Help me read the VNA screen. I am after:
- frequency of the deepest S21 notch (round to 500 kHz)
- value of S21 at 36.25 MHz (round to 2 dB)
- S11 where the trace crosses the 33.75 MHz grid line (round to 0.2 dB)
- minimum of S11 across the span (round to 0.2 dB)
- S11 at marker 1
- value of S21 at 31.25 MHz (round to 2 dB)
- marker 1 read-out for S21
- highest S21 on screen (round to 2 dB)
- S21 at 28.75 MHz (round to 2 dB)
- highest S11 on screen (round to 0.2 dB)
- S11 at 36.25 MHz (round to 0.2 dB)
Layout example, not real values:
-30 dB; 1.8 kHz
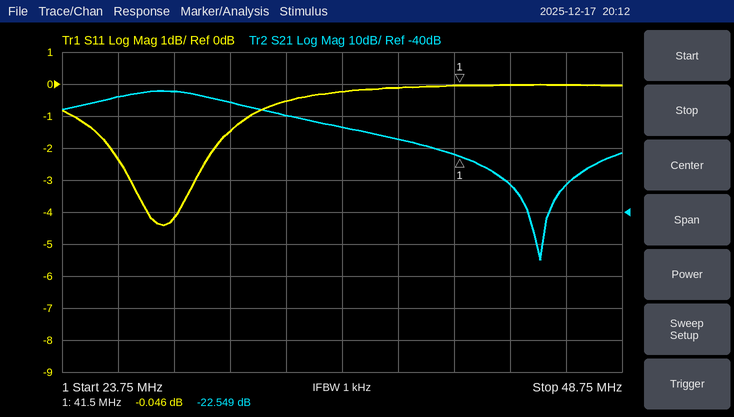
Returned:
45.0 MHz; -14 dB; -0.6 dB; -4.4 dB; -0.046 dB; -6 dB; -22.549 dB; -2 dB; -2 dB; 0.0 dB; -0.2 dB
